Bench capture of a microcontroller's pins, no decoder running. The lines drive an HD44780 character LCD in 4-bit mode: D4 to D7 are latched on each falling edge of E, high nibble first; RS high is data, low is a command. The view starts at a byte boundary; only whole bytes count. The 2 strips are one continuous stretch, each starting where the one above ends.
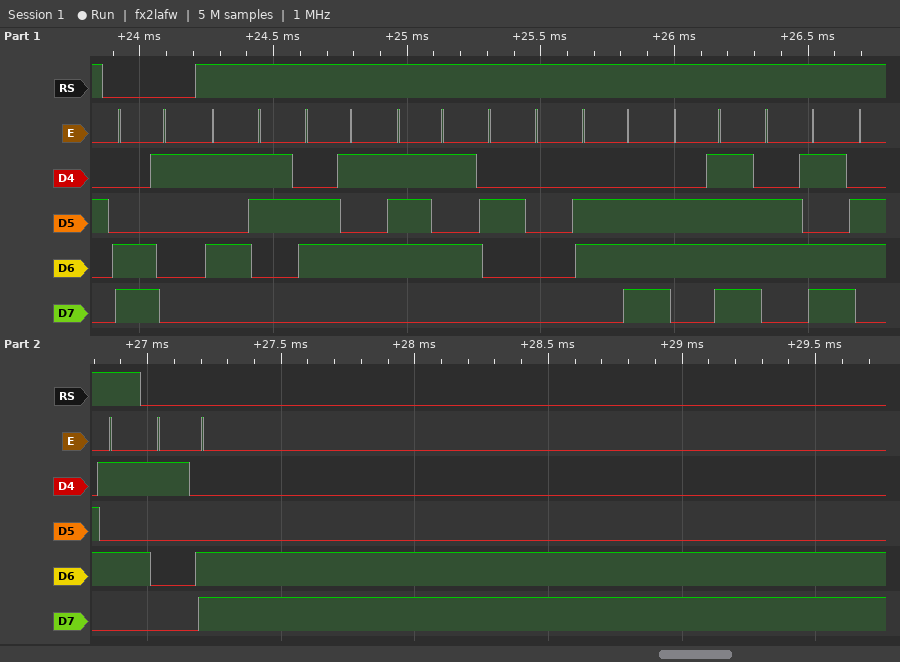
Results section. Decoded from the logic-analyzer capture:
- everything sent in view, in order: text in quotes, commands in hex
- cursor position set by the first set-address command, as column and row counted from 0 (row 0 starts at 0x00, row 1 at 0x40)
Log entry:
0xC1 "Seu nome" 0x1C
column 1, row 1
